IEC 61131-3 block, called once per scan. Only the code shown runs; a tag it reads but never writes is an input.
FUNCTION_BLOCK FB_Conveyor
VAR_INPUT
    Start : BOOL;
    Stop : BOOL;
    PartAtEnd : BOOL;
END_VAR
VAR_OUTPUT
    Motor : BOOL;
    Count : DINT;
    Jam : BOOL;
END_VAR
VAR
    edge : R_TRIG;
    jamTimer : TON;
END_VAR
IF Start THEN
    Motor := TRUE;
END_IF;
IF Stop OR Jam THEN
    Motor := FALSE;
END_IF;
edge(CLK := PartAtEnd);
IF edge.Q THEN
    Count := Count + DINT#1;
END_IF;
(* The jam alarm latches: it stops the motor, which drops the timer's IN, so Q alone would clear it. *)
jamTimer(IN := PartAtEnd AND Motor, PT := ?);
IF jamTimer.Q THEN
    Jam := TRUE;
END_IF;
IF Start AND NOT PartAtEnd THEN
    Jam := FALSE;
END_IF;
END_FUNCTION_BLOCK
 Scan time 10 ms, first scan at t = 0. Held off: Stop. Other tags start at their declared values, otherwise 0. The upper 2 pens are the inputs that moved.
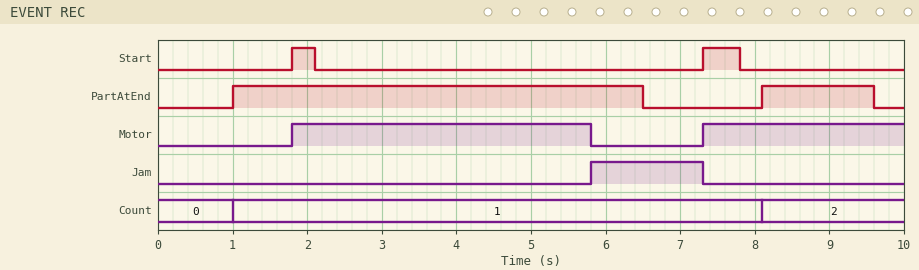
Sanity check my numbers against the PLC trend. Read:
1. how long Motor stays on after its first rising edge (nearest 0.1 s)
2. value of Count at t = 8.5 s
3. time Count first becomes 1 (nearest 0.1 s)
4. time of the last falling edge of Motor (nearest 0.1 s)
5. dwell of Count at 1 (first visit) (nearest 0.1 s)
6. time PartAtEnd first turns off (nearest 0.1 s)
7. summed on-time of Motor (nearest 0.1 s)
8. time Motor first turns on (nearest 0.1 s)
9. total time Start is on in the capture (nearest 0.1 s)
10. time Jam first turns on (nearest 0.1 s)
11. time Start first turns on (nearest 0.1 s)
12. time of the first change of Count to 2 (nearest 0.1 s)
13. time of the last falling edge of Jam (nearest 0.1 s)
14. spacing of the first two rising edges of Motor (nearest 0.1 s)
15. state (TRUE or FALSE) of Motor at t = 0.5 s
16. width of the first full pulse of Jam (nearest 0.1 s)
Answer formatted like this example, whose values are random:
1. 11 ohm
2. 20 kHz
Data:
1. 4.0 s
2. 2
3. 1.0 s
4. 5.8 s
5. 7.1 s
6. 6.5 s
7. 6.7 s
8. 1.8 s
9. 0.8 s
10. 5.8 s
11. 1.8 s
12. 8.1 s
13. 7.3 s
14. 5.5 s
15. FALSE
16. 1.5 s
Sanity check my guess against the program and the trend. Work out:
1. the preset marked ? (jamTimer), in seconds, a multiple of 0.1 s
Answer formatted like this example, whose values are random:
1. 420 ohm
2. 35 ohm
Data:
1. 4.0 s
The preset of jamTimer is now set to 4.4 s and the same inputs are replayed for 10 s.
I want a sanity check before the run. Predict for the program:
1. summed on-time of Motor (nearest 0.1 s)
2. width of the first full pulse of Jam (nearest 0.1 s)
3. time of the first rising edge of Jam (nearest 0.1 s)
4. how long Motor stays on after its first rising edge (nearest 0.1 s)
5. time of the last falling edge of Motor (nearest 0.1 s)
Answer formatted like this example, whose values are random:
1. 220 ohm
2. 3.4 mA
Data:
1. 7.1 s
2. 1.1 s
3. 6.2 s
4. 4.4 s
5. 6.2 s
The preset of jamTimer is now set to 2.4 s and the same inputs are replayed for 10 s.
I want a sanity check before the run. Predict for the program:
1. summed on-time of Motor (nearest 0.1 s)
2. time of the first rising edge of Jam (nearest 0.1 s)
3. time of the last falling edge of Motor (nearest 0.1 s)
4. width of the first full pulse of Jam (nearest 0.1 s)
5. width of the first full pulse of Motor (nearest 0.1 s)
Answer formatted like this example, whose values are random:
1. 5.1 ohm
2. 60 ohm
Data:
1. 5.1 s
2. 4.2 s
3. 4.2 s
4. 3.1 s
5. 2.4 s
